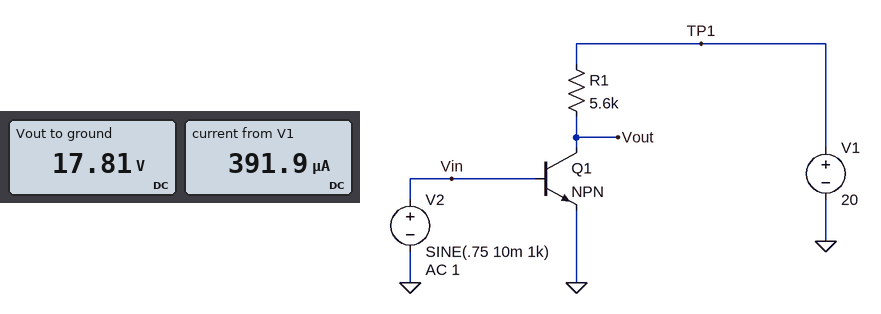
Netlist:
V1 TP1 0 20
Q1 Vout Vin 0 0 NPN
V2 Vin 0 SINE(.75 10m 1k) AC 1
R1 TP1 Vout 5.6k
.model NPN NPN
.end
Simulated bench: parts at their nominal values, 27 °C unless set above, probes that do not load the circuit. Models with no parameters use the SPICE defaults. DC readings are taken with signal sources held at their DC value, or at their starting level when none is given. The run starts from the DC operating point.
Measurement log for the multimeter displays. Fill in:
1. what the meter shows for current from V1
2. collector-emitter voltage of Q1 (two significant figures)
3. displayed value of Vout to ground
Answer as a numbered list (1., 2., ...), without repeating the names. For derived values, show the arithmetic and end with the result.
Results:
1. 391.9 µA
2. 17.81 V = 18 V
3. 17.81 V
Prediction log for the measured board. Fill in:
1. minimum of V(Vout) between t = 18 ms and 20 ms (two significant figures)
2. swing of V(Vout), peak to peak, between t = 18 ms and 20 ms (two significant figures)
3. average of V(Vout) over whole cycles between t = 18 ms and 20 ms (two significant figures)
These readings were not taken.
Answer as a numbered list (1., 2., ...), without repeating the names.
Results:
1. 17 V
2. 1.7 V
3. 18 V
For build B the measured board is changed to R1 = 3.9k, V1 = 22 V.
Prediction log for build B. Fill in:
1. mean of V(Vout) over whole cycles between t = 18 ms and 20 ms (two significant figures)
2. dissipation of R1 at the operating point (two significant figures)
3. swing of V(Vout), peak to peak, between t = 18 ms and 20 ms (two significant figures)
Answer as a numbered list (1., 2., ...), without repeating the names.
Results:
1. 20 V
2. 600 µW
3. 1.2 V
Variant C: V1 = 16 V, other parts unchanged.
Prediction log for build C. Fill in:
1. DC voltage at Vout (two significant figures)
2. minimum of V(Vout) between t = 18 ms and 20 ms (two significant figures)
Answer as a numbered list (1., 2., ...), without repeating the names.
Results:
1. 14 V
2. 13 V
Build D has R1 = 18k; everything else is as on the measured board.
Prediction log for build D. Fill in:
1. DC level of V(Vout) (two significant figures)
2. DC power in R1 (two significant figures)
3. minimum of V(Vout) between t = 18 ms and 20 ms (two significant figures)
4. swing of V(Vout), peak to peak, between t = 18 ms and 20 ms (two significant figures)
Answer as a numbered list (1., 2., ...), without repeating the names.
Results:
1. 13 V
2. 2.8 mW
3. 9.6 V
4. 5.6 V
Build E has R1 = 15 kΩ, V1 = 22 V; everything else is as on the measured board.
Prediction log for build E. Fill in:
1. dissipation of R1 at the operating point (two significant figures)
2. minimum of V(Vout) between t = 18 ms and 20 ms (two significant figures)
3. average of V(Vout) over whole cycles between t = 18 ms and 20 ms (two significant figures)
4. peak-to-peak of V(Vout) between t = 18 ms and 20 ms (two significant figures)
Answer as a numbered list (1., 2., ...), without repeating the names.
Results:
1. 2.3 mW
2. 13 V
3. 16 V
4. 4.7 V
